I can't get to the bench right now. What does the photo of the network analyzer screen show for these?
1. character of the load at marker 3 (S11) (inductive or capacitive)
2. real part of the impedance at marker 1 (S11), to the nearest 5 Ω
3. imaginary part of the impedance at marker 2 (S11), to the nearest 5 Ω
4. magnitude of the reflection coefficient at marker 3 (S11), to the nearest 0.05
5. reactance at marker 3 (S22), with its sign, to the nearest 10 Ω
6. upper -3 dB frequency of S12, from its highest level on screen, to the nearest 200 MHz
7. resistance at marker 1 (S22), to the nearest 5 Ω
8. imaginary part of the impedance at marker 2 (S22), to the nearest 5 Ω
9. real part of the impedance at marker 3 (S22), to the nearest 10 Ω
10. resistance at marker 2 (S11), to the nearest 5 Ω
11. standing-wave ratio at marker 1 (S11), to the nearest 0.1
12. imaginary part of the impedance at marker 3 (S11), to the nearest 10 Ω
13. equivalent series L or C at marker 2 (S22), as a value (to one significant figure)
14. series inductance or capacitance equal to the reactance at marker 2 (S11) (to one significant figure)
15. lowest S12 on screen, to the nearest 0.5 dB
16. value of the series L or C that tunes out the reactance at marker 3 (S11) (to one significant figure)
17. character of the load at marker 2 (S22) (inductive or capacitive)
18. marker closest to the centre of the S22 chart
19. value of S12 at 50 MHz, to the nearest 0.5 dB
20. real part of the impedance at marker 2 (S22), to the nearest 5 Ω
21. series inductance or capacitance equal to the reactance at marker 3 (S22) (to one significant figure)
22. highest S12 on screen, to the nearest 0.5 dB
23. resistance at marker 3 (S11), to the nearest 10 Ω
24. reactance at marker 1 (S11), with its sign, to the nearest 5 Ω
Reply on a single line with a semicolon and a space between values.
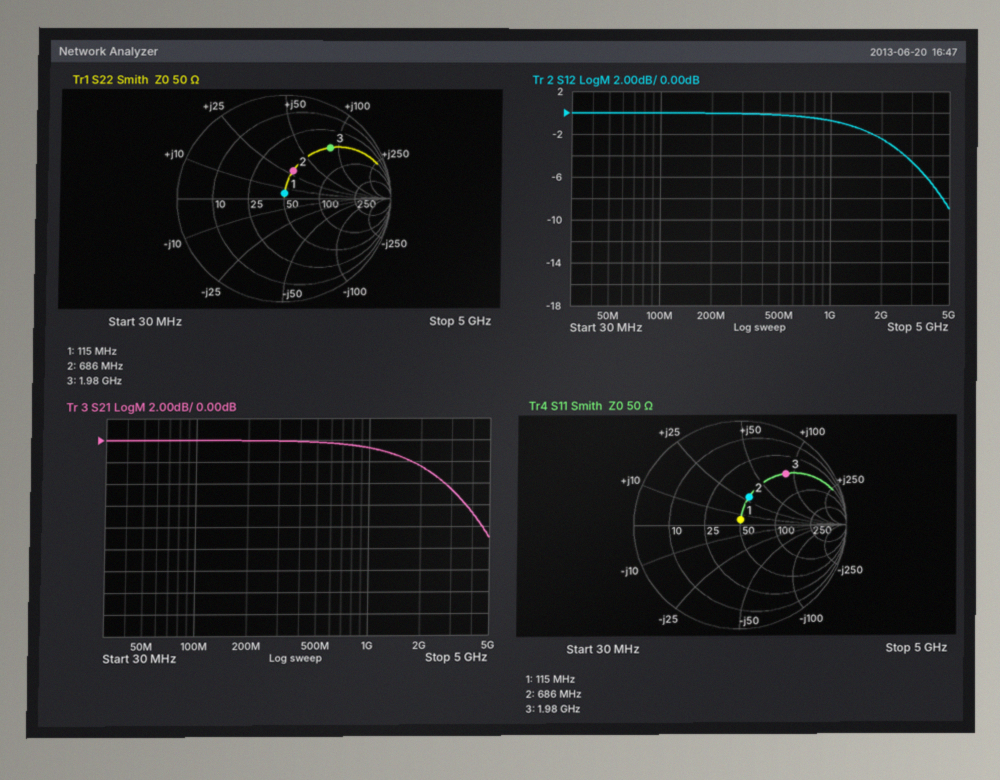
inductive; 50 Ω; +30 Ω; 0.65; +90 Ω; 2.2 GHz; 50 Ω; +30 Ω; 50 Ω; 50 Ω; 1.1; +90 Ω; 7 nH; 7 nH; -9.0 dB; 900 fF; inductive; marker 1; 0.0 dB; 50 Ω; 7 nH; 0.0 dB; 50 Ω; +5 Ω
